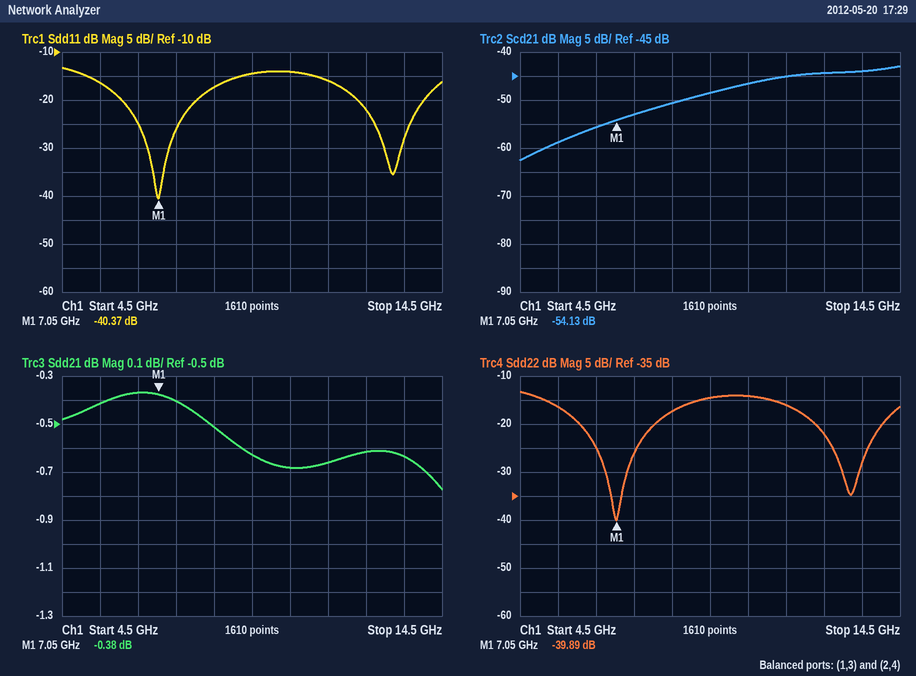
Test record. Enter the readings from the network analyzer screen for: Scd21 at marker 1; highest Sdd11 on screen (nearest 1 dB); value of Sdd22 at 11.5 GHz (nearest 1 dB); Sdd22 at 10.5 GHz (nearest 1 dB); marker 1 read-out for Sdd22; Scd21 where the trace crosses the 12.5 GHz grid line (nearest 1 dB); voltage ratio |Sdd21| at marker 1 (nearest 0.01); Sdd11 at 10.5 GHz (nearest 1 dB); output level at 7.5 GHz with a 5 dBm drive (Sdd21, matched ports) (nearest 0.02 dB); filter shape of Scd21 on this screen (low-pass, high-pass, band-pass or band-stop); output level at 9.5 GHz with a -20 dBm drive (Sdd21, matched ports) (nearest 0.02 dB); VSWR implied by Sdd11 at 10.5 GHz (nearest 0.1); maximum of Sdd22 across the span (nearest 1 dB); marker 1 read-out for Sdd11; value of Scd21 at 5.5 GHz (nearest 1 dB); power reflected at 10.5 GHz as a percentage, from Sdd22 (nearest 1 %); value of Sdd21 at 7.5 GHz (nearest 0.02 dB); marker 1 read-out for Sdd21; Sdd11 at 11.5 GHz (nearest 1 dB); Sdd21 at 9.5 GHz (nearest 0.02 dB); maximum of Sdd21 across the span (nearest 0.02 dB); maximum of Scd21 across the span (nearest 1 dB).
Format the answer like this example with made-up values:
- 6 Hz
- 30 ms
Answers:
- -54.13 dB
- -13 dB
- -16 dB
- -14 dB
- -39.89 dB
- -44 dB
- 0.96
- -14 dB
- 4.60 dBm
- high-pass
- -20.62 dBm
- 1.5
- -13 dB
- -40.37 dB
- -59 dB
- 4 %
- -0.40 dB
- -0.38 dB
- -16 dB
- -0.62 dB
- -0.36 dB
- -43 dB
